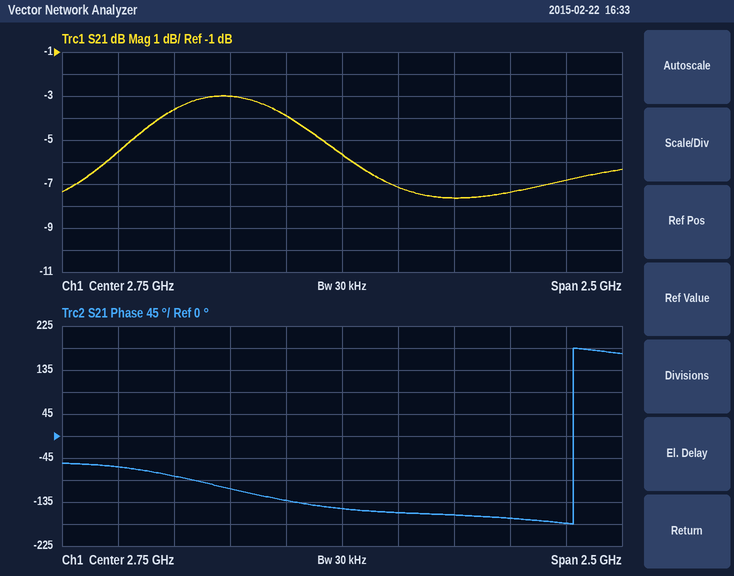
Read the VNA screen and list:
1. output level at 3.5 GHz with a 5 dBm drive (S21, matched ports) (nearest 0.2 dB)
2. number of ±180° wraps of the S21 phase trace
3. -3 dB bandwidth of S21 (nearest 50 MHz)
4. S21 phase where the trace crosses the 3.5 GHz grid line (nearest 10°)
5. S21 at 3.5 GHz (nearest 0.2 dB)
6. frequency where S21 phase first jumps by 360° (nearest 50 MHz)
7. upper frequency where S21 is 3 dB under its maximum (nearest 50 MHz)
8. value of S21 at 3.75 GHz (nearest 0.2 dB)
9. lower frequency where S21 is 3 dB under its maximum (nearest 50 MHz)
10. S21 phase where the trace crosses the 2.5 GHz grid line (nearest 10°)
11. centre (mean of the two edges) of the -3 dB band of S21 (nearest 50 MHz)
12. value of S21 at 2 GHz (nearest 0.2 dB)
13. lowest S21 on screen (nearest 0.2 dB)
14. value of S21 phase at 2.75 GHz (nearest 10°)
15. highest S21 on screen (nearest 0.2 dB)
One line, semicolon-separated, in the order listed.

-2.4 dBm; 1; 1.10 GHz; -170°; -7.4 dB; 3.80 GHz; 2.80 GHz; -6.8 dB; 1.70 GHz; -130°; 2.25 GHz; -3.6 dB; -7.6 dB; -150°; -3.0 dB
